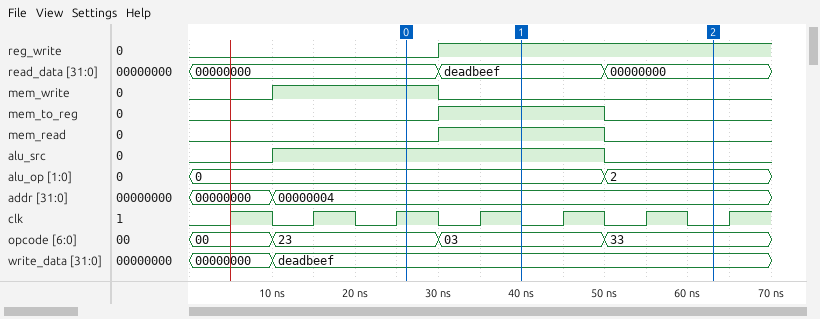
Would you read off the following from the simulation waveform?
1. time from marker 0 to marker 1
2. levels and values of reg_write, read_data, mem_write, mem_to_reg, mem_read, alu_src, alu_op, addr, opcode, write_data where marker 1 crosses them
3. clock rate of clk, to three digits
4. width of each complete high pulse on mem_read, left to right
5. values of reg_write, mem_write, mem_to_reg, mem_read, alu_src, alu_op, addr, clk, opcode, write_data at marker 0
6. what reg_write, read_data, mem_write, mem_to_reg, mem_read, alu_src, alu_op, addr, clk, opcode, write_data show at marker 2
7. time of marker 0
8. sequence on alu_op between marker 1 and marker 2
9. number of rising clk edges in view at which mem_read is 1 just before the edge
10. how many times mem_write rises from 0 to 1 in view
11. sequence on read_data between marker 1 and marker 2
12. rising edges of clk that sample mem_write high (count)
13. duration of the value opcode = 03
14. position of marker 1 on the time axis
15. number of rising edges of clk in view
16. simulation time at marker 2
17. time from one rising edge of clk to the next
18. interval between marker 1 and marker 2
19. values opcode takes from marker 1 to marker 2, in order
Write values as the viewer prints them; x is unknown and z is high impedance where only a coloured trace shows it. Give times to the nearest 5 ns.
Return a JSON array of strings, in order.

["15 ns", "reg_write=1, read_data=deadbeef, mem_write=0, mem_to_reg=1, mem_read=1, alu_src=1, alu_op=0, addr=00000004, opcode=03, write_data=deadbeef", "100 MHz", "20 ns", "reg_write=0, mem_write=1, mem_to_reg=0, mem_read=0, alu_src=1, alu_op=0, addr=00000004, clk=1, opcode=23, write_data=deadbeef", "reg_write=1, read_data=00000000, mem_write=0, mem_to_reg=0, mem_read=0, alu_src=0, alu_op=2, addr=00000004, clk=0, opcode=33, write_data=deadbeef", "25 ns", "0, 2", "2", "1", "deadbeef, 00000000", "2", "20 ns", "40 ns", "7", "65 ns", "10 ns", "25 ns", "03, 33"]
